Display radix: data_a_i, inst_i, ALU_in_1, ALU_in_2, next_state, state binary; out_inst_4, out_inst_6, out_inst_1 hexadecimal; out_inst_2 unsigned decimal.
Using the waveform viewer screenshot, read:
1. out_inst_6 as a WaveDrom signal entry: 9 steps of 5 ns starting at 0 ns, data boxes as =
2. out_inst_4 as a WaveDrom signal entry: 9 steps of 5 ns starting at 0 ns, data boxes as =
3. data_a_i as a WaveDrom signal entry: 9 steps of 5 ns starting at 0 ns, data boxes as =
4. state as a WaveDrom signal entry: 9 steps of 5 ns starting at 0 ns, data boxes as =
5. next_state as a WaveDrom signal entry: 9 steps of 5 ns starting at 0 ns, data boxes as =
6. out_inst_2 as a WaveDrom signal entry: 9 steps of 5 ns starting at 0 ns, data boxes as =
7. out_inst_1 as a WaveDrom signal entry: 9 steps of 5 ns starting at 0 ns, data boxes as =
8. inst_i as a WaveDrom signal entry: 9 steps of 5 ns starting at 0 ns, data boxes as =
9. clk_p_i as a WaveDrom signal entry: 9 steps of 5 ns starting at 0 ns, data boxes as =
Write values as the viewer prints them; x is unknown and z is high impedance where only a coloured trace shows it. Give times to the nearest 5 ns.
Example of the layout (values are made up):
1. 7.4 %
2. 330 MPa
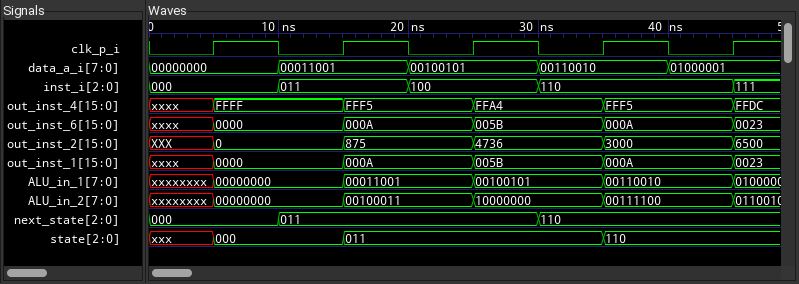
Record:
1. {name: 'out_inst_6', wave: 'x=.=.=.=.', data: '0000 000A 005B 000A'}
2. {name: 'out_inst_4', wave: 'x=.=.=.=.', data: 'FFFF FFF5 FFA4 FFF5'}
3. {name: 'data_a_i', wave: '=.=.=.=.=', data: '00000000 00011001 00100101 00110010 01000001'}
4. {name: 'state', wave: 'x=.=...=.', data: '000 011 110'}
5. {name: 'next_state', wave: '=.=...=..', data: '000 011 110'}
6. {name: 'out_inst_2', wave: 'x=.=.=.=.', data: '0 875 4736 3000'}
7. {name: 'out_inst_1', wave: 'x=.=.=.=.', data: '0000 000A 005B 000A'}
8. {name: 'inst_i', wave: '=.=.=.=..', data: '000 011 100 110'}
9. {name: 'clk_p_i', wave: '010101010'}
